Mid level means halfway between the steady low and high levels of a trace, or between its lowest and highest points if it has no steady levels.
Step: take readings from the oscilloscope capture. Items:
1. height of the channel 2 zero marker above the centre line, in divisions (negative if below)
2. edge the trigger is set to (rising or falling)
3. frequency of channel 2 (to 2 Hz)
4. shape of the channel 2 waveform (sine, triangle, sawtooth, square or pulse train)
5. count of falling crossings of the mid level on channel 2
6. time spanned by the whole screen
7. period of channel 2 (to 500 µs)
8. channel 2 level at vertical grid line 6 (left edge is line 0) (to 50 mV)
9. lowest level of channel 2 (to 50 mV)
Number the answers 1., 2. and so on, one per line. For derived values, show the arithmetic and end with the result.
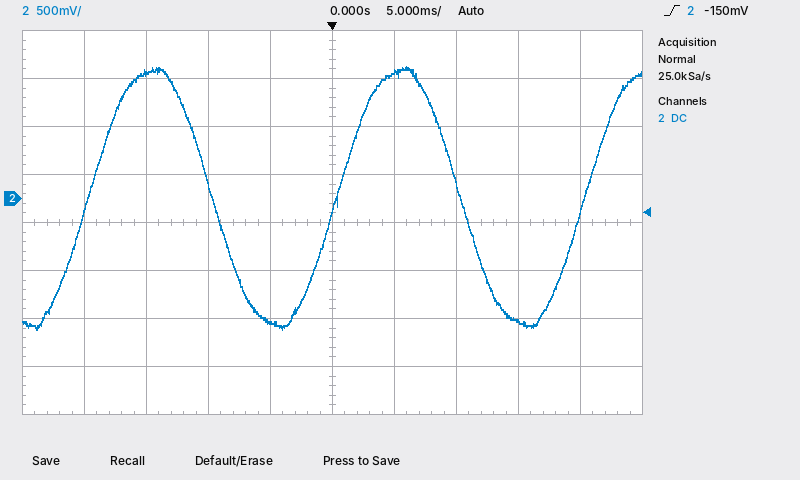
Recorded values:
1. +0.5 div
2. rising
3. 1 / 20.0 ms ≈ 50 Hz
4. sine
5. 2
6. 50 ms
7. 20.0 ms
8. 1.30 V
9. -1.35 V
